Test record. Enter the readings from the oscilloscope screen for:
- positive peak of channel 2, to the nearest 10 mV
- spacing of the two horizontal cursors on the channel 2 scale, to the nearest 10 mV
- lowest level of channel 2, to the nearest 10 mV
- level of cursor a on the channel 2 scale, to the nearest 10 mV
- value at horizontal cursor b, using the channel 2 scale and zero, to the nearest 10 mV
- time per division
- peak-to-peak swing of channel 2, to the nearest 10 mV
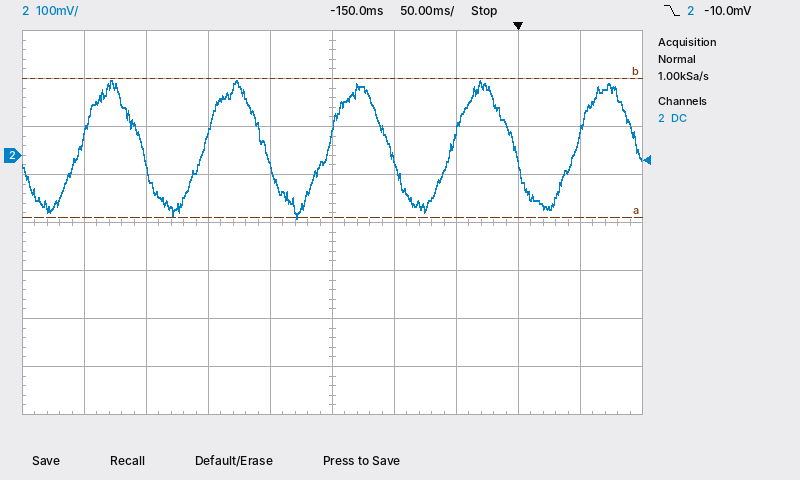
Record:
160 mV
290 mV
-130 mV
-130 mV
160 mV
50 ms
290 mV
